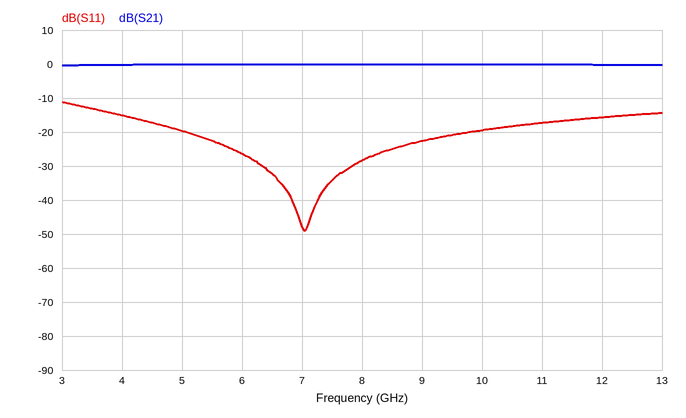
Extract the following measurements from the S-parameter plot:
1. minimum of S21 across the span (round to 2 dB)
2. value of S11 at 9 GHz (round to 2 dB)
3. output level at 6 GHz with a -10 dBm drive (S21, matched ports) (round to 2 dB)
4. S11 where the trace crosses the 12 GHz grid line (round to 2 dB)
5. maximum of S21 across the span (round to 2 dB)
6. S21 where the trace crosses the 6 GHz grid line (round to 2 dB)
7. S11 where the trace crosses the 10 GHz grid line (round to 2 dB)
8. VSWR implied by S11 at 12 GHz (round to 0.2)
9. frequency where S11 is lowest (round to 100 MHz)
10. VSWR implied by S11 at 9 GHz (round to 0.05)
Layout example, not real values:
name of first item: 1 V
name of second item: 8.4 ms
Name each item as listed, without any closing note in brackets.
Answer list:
minimum of S21 across the span: 0 dB
value of S11 at 9 GHz: -22 dB
output level at 6 GHz with a -10 dBm drive (S21, matched ports): -10 dBm
S11 where the trace crosses the 12 GHz grid line: -16 dB
maximum of S21 across the span: 0 dB
S21 where the trace crosses the 6 GHz grid line: 0 dB
S11 where the trace crosses the 10 GHz grid line: -20 dB
VSWR implied by S11 at 12 GHz: 1.4
frequency where S11 is lowest: 7.0 GHz
VSWR implied by S11 at 9 GHz: 1.15
